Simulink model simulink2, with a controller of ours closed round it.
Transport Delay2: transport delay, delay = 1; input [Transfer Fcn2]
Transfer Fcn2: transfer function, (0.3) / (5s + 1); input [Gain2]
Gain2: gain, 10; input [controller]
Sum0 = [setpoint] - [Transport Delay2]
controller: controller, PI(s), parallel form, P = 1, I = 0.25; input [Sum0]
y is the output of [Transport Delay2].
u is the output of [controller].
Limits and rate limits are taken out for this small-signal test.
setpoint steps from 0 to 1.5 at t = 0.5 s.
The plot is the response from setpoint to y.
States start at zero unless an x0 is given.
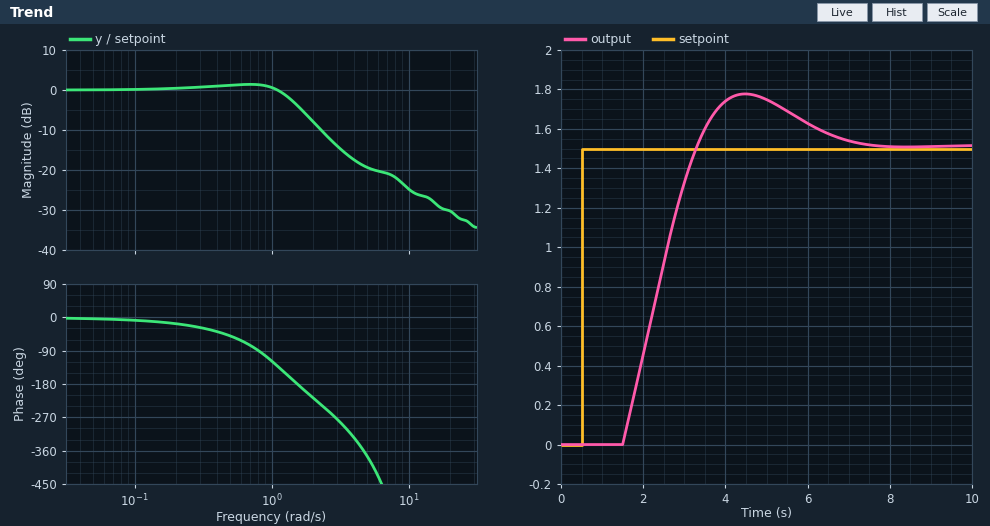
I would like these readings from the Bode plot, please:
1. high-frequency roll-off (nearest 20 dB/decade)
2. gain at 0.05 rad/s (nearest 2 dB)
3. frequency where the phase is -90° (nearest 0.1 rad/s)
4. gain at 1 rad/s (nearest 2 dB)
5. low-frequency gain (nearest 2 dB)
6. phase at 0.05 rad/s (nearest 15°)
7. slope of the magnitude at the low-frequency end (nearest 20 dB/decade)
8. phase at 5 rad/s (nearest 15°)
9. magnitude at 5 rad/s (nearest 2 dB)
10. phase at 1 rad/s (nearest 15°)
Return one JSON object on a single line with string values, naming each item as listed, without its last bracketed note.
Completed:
{"high-frequency roll-off": "-20 dB/decade", "gain at 0.05 rad/s": "0 dB", "frequency where the phase is -90°": "0.8 rad/s", "gain at 1 rad/s": "0 dB", "low-frequency gain": "0 dB", "phase at 0.05 rad/s": "0°", "slope of the magnitude at the low-frequency end": "0 dB/decade", "phase at 5 rad/s": "-375°", "magnitude at 5 rad/s": "-20 dB", "phase at 1 rad/s": "-120°"}
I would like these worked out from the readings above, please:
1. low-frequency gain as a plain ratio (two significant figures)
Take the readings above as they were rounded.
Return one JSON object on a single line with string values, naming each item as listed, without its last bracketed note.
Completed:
{"low-frequency gain as a plain ratio": "1.0"}
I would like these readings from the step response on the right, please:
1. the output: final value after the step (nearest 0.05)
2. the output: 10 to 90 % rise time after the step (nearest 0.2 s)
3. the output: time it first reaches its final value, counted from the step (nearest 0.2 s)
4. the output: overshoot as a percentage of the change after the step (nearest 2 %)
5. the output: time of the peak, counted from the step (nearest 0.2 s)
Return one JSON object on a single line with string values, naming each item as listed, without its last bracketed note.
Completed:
{"the output: final value after the step": "1.50", "the output: 10 to 90 % rise time after the step": "1.4 s", "the output: time it first reaches its final value, counted from the step": "2.8 s", "the output: overshoot as a percentage of the change after the step": "18 %", "the output: time of the peak, counted from the step": "4.0 s"}
